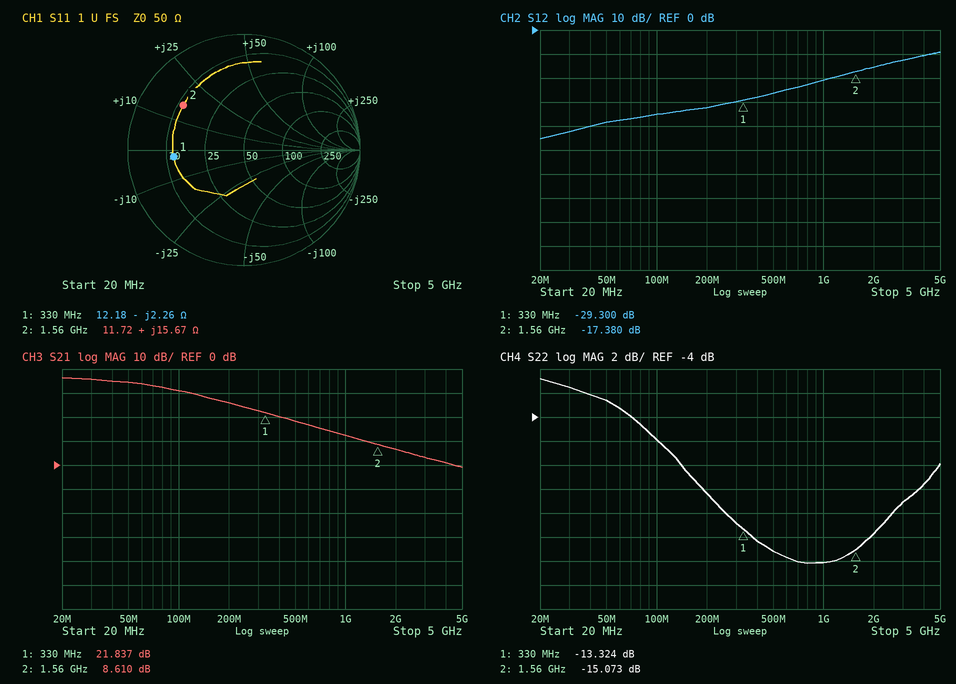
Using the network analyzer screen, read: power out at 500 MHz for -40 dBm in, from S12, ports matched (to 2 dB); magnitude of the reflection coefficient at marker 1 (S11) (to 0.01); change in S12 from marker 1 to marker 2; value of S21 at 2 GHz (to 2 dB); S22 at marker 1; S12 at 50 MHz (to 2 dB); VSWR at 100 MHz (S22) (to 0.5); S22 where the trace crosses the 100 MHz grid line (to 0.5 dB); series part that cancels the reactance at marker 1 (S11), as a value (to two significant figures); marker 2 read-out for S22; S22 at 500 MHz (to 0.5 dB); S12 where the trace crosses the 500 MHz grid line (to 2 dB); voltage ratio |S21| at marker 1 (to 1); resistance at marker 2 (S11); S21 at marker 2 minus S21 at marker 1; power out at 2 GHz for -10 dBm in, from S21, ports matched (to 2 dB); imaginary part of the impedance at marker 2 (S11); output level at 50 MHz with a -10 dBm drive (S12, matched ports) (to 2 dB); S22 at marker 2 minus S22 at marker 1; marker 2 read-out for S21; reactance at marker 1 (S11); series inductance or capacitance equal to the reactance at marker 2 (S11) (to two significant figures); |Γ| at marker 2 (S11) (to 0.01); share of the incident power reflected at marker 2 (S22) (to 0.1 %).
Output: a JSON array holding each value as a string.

["-66 dBm", "0.61", "11.920 dB", "6 dB", "-13.324 dB", "-38 dB", "3.0", "-6.0 dB", "1.1 nH", "-15.073 dB", "-15.0 dB", "-26 dB", "12", "11.72 Ω", "-13.227 dB", "-4 dBm", "+15.67 Ω", "-48 dBm", "-1.749 dB", "8.610 dB", "-2.26 Ω", "1.6 nH", "0.65", "3.1 %"]
